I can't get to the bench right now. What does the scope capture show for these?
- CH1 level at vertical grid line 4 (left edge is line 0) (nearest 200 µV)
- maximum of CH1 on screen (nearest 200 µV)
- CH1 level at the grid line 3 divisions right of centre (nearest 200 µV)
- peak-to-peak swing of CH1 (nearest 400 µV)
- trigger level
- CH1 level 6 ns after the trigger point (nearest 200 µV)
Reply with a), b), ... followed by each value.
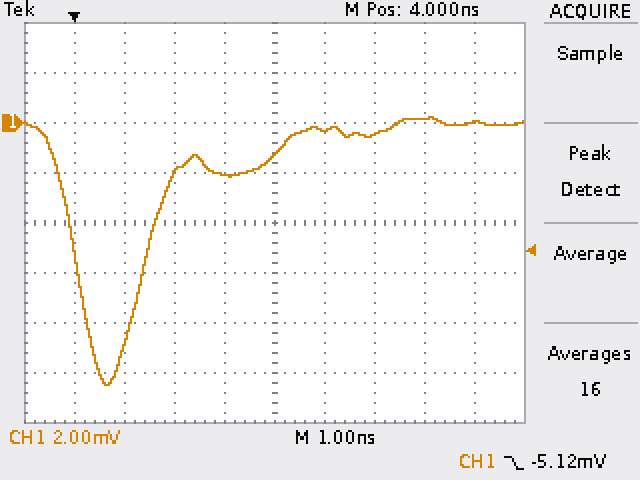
a) -2.0 mV
b) 200 µV
c) 200 µV
d) 10.8 mV
e) -5.12 mV
f) -400 µV
